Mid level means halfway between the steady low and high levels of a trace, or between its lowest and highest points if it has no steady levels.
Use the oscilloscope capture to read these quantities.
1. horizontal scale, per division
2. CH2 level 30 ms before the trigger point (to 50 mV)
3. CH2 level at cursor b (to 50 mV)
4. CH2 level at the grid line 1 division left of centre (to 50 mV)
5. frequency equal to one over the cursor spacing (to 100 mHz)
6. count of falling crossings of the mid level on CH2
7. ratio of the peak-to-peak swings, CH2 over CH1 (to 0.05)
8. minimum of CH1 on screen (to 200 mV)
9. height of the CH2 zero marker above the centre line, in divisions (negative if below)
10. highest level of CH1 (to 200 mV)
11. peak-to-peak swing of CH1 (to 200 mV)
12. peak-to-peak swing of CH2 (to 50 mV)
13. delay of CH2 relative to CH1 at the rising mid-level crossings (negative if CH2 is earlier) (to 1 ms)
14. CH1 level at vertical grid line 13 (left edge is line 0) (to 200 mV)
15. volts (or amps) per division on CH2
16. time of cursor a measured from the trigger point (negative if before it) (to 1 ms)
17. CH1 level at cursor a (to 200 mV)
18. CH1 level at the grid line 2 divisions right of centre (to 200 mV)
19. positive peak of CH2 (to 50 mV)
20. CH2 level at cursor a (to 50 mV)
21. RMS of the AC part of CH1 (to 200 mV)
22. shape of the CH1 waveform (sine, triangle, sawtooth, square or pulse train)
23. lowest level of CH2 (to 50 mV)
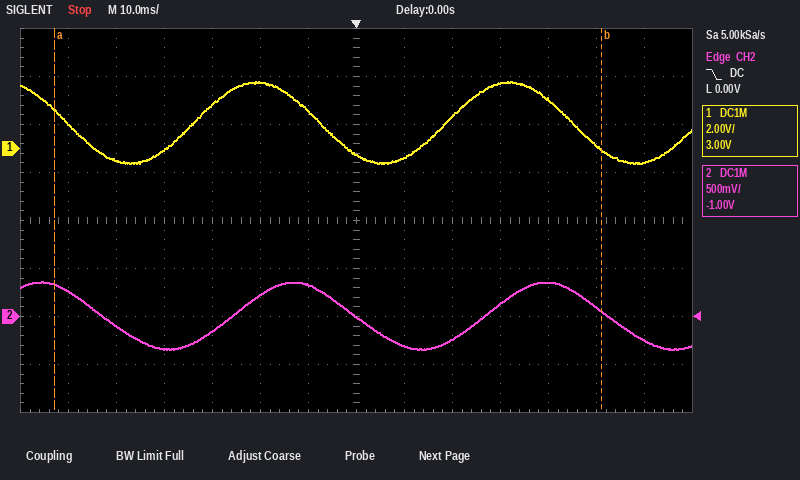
10 ms
-150 mV
50 mV
350 mV
8.8 Hz
3
0.20
-600 mV
-2.0 div
2.8 V
3.4 V
700 mV
+8 ms
-600 mV
500 mV
-63 ms
1.6 V
1.4 V
350 mV
350 mV
1.2 V
sine
-350 mV
